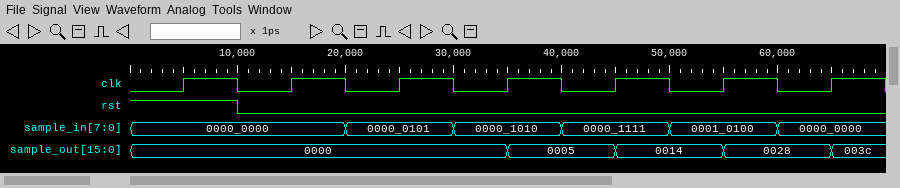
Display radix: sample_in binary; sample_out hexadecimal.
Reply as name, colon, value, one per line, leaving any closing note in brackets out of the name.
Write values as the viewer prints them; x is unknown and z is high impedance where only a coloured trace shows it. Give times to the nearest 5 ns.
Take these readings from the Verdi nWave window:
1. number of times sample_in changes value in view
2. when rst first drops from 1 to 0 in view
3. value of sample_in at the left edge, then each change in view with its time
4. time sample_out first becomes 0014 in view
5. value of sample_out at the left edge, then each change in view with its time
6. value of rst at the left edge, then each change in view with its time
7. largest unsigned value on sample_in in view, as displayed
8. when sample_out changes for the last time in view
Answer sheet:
number of times sample_in changes value in view: 5
when rst first drops from 1 to 0 in view: 10 ns
value of sample_in at the left edge, then each change in view with its time: 0000_0000, 0000_0101 at 20 ns, 0000_1010 at 30 ns, 0000_1111 at 40 ns, 0001_0100 at 50 ns, 0000_0000 at 60 ns
time sample_out first becomes 0014 in view: 45 ns
value of sample_out at the left edge, then each change in view with its time: 0000, 0005 at 35 ns, 0014 at 45 ns, 0028 at 55 ns, 003c at 65 ns
value of rst at the left edge, then each change in view with its time: 1, 0 at 10 ns
largest unsigned value on sample_in in view, as displayed: 0001_0100
when sample_out changes for the last time in view: 65 ns
